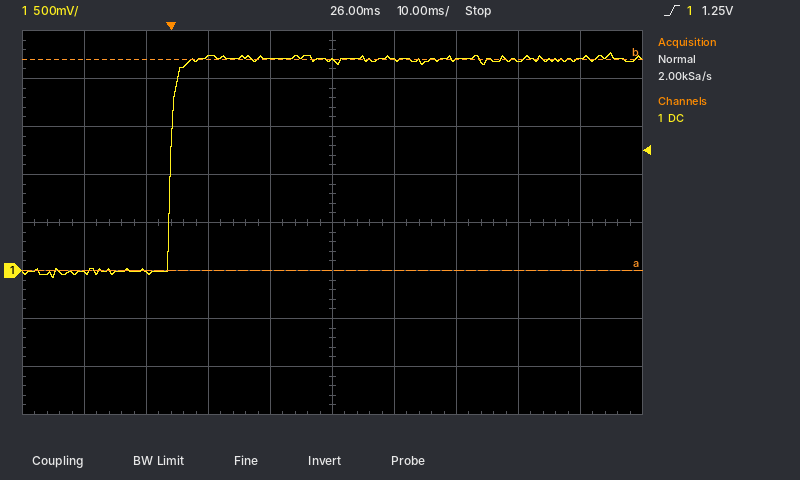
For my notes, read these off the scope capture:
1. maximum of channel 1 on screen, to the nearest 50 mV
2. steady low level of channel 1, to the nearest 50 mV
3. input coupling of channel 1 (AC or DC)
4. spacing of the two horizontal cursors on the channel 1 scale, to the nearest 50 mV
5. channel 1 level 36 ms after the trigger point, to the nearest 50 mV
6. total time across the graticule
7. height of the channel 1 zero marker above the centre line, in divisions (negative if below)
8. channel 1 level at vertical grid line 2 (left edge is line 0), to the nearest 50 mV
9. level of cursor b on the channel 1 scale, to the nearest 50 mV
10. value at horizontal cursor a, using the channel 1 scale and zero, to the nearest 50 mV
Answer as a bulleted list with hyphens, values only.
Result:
- 2.25 V
- 0 mV
- DC
- 2.20 V
- 2.20 V
- 100 ms
- -1.0 div
- 0 mV
- 2.20 V
- 0 mV
